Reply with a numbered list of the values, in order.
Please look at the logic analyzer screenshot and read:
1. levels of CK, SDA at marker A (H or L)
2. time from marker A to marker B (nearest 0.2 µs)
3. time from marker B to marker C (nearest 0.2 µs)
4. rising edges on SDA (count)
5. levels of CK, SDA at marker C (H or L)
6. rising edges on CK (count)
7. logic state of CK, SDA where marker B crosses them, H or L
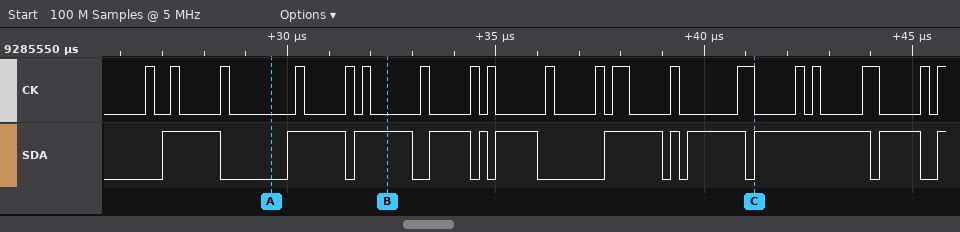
1. CK=L, SDA=L
2. 2.8 µs
3. 8.8 µs
4. 12
5. CK=L, SDA=H
6. 19
7. CK=L, SDA=H
